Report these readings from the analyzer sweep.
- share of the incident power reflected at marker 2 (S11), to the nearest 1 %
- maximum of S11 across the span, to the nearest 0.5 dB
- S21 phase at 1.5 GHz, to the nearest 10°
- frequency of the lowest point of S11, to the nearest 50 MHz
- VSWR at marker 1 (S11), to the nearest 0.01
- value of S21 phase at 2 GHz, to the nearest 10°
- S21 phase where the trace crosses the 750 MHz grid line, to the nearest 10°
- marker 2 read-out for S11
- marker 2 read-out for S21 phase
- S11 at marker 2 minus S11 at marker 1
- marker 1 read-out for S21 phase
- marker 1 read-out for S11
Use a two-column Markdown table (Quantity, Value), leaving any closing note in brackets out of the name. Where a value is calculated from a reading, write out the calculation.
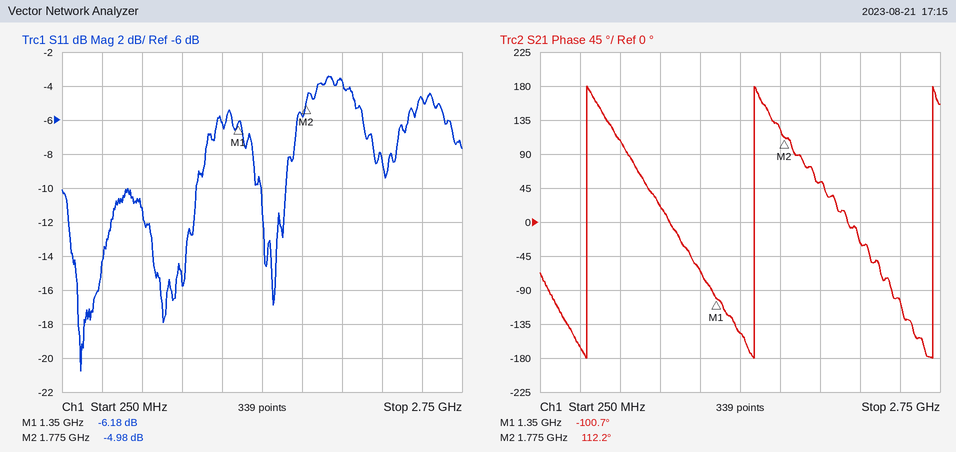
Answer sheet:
| Quantity | Value |
|---|---|
| share of the incident power reflected at marker 2 (S11), to the nearest 1 % | 10^(-4.98/10) ≈ 32 % |
| maximum of S11 across the span, to the nearest 0.5 dB | -3.5 dB |
| S21 phase at 1.5 GHz, to the nearest 10° | -150° |
| frequency of the lowest point of S11, to the nearest 50 MHz | 350 MHz |
| VSWR at marker 1 (S11), to the nearest 0.01 | (1 + 0.4909)/(1 − 0.4909) ≈ 2.93 |
| value of S21 phase at 2 GHz, to the nearest 10° | 50° |
| S21 phase where the trace crosses the 750 MHz grid line, to the nearest 10° | 110° |
| marker 2 read-out for S11 | -4.98 dB |
| marker 2 read-out for S21 phase | 112.2° |
| S11 at marker 2 minus S11 at marker 1 | -4.98 − (-6.18) = 1.20 dB |
| marker 1 read-out for S21 phase | -100.7° |
| marker 1 read-out for S11 | -6.18 dB |
